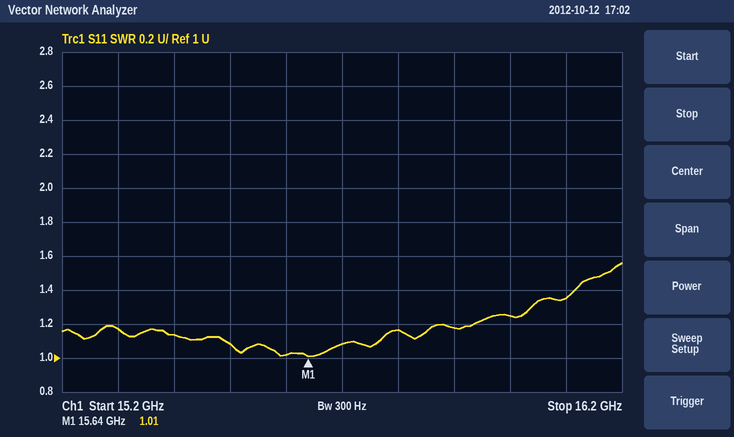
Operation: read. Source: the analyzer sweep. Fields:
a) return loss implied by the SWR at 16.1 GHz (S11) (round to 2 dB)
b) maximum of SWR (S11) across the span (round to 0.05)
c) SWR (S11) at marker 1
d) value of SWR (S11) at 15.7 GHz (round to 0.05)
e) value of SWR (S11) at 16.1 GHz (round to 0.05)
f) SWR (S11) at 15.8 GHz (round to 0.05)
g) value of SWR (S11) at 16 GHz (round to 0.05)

16 dB
1.55
1.01
1.10
1.35
1.15
1.25
